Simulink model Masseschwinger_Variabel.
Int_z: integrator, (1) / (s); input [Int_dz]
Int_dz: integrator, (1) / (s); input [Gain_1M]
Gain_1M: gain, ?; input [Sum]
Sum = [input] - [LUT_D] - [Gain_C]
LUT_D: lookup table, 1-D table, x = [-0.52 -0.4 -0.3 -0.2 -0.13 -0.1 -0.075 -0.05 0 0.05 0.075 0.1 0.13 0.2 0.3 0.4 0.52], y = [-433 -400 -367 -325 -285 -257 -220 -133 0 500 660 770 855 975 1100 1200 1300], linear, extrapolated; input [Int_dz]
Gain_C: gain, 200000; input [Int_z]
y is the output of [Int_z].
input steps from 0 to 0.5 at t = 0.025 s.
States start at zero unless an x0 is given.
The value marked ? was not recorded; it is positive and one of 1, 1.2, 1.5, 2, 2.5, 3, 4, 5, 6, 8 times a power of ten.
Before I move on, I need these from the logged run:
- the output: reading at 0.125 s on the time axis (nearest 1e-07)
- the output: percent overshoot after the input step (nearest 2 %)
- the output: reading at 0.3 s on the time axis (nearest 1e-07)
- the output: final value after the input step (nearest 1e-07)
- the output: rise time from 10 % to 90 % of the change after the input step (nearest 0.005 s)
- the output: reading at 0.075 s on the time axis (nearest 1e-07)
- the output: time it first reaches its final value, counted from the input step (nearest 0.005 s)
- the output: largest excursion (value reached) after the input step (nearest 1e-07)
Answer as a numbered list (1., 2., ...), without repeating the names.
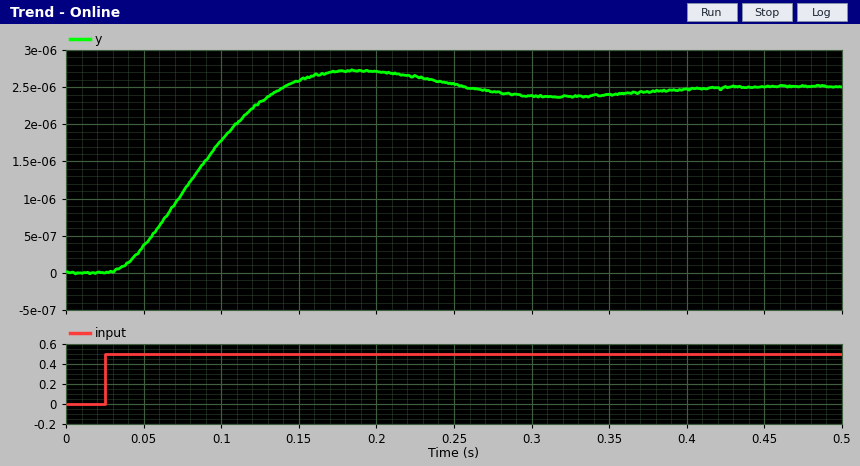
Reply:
1. 0.0000023
2. 8 %
3. 0.0000024
4. 0.0000025
5. 0.075 s
6. 0.0000011
7. 0.115 s
8. 0.0000027
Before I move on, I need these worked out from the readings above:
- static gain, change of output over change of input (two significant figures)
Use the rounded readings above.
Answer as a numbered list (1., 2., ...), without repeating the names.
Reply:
1. 0.0000050
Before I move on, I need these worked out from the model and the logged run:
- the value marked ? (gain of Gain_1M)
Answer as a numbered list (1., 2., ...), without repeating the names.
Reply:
1. 0.003
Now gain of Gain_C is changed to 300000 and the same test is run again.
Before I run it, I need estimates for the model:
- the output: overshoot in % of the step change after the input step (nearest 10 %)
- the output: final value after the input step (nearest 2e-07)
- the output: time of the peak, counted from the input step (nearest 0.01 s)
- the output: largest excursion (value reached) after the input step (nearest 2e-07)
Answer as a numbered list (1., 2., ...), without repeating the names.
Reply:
1. 20 %
2. 0.0000016
3. 0.12 s
4. 0.0000020
